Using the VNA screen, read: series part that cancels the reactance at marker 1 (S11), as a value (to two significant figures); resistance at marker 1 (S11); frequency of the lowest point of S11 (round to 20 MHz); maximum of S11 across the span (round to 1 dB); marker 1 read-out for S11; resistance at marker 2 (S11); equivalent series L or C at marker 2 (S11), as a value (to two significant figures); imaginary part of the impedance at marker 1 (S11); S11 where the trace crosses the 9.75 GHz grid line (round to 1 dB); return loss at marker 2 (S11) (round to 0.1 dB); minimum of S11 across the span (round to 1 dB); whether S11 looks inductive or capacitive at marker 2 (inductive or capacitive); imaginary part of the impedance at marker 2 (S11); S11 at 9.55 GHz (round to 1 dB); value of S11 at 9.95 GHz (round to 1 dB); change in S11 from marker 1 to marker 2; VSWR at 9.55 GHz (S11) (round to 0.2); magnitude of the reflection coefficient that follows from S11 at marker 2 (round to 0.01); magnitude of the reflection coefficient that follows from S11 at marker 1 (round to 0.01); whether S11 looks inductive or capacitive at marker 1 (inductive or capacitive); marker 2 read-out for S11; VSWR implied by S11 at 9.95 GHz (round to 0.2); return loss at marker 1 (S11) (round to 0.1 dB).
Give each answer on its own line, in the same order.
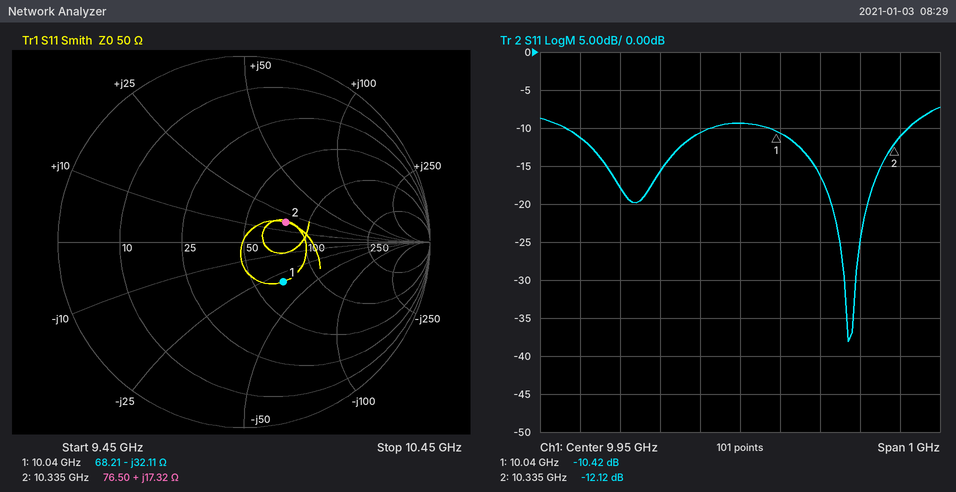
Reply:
510 pH
68.21 Ω
10.22 GHz
-7 dB
-10.42 dB
76.50 Ω
270 pH
-32.11 Ω
-16 dB
12.1 dB
-38 dB
inductive
+17.32 Ω
-11 dB
-9 dB
-1.70 dB
1.8
0.25
0.30
capacitive
-12.12 dB
2.0
10.4 dB
